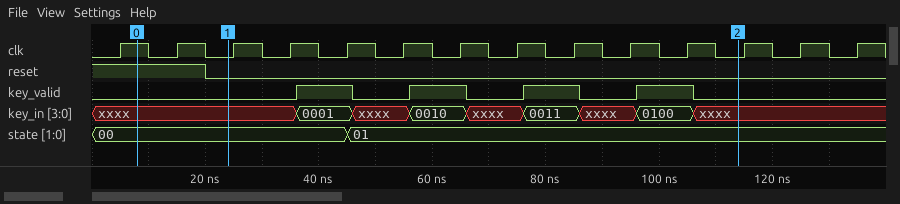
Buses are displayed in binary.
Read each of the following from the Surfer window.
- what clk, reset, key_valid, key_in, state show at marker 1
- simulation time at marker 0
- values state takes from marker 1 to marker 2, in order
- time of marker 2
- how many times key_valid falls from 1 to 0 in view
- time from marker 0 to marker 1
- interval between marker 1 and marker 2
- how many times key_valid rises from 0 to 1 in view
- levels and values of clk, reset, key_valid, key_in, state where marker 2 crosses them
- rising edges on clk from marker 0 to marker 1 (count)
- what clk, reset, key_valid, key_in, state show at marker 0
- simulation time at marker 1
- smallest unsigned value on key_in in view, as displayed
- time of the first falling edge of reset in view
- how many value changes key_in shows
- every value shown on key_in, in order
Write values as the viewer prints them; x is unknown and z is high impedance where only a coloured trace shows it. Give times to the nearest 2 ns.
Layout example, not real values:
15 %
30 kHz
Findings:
clk=0, reset=0, key_valid=0, key_in=xxxx, state=00
8 ns
00, 01
114 ns
4
16 ns
90 ns
4
clk=0, reset=0, key_valid=0, key_in=xxxx, state=01
1
clk=1, reset=1, key_valid=0, key_in=xxxx, state=00
24 ns
0001
20 ns
8
xxxx, 0001, xxxx, 0010, xxxx, 0011, xxxx, 0100, xxxx
